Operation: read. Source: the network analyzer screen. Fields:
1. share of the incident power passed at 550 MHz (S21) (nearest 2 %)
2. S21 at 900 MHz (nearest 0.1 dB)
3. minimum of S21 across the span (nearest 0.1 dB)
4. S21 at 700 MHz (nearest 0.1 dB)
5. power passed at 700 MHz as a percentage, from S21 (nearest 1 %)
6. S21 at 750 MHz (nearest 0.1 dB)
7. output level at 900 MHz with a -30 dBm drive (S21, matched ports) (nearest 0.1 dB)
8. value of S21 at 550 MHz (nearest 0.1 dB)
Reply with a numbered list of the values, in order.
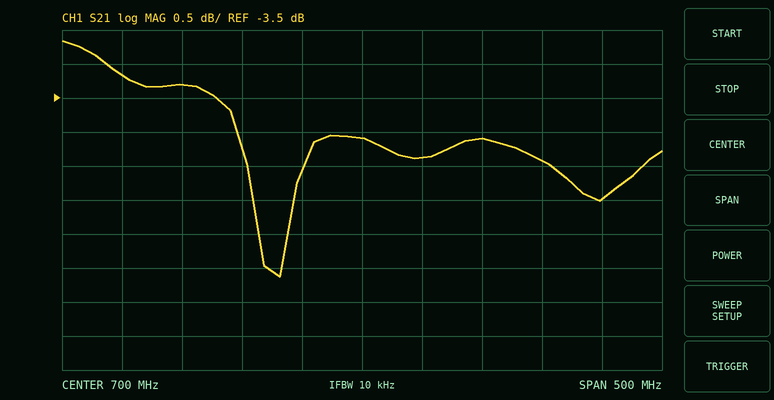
1. 46 %
2. -5.0 dB
3. -6.1 dB
4. -4.1 dB
5. 39 %
6. -4.4 dB
7. -35.0 dBm
8. -3.3 dB
